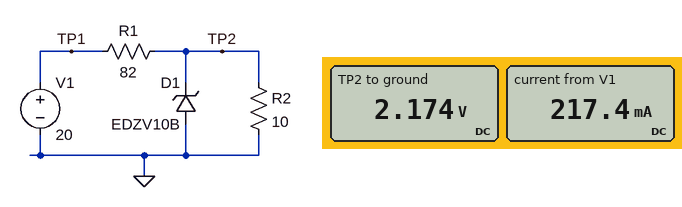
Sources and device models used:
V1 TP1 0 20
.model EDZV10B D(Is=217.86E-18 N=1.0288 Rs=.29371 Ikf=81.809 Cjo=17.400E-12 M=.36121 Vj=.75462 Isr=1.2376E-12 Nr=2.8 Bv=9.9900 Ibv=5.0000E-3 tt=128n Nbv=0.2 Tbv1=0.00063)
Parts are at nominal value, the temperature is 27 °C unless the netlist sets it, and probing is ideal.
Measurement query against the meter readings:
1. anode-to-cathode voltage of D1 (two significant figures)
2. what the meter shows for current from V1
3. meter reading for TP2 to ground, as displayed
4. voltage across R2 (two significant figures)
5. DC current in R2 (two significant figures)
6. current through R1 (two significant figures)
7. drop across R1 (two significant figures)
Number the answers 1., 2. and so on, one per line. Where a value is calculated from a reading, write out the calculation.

1. 0 V - 2.174 V = -2.2 V
2. 217.4 mA
3. 2.174 V
4. 2.174 V = 2.2 V
5. (2.174 V) / 10 Ω = 220 mA
6. (20 V - 2.174 V) / 82 Ω = 220 mA
7. 20 V - 2.174 V = 18 V
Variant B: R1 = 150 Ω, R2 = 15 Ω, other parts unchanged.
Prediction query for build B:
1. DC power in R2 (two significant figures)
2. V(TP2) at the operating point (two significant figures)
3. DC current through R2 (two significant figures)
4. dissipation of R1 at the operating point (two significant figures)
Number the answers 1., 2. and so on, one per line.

1. 220 mW
2. 1.8 V
3. 120 mA
4. 2.2 W
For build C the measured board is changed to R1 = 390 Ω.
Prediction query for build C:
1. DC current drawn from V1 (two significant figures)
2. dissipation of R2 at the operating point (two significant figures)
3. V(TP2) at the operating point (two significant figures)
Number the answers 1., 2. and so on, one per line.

1. 50 mA
2. 25 mW
3. 500 mV
